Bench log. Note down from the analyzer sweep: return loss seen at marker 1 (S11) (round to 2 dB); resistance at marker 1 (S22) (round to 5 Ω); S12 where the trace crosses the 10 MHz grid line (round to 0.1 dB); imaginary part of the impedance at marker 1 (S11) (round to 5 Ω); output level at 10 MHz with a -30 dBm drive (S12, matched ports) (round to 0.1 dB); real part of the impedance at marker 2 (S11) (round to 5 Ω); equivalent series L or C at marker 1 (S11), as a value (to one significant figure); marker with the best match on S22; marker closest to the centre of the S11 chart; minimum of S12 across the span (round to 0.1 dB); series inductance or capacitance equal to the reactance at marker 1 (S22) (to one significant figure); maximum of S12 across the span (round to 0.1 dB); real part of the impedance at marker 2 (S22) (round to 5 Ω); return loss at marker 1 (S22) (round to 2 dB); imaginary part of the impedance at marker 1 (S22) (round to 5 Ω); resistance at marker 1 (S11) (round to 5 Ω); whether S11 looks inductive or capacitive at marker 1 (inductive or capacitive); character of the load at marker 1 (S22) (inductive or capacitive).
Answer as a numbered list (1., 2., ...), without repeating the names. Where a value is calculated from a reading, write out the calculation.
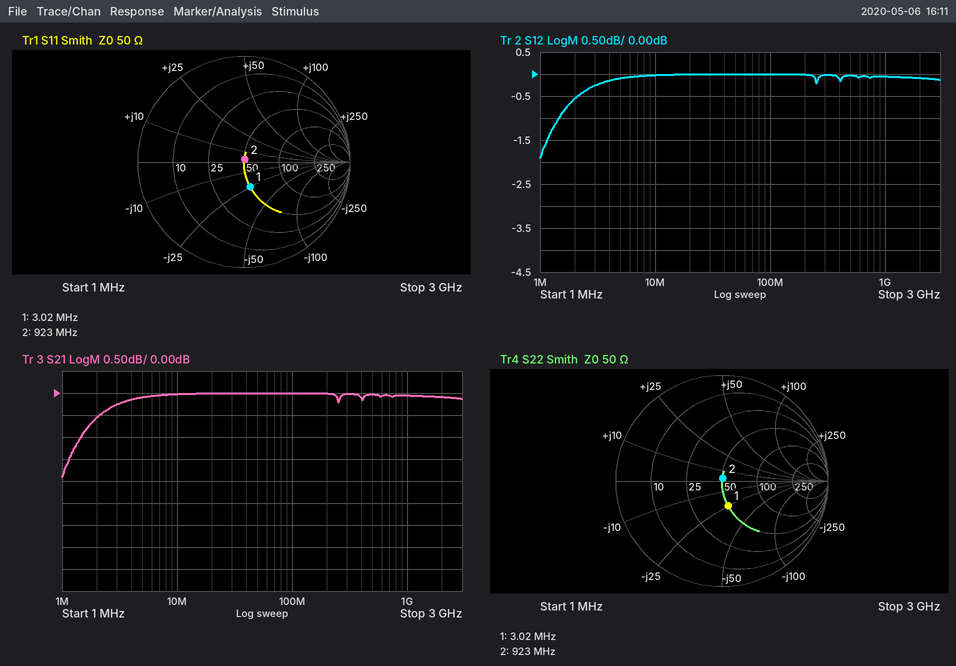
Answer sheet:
1. 12 dB
2. 50 Ω
3. 0.0 dB
4. -25 Ω
5. -30 dBm + (0.0 dB) = -30.0 dBm
6. 50 Ω
7. C = 1/(2π × 3.02 MHz × 25 Ω) ≈ 2 nF
8. marker 2
9. marker 2
10. -1.9 dB
11. C = 1/(2π × 3.02 MHz × 25 Ω) ≈ 2 nF
12. 0.0 dB
13. 50 Ω
14. 12 dB
15. -25 Ω
16. 50 Ω
17. capacitive
18. capacitive
